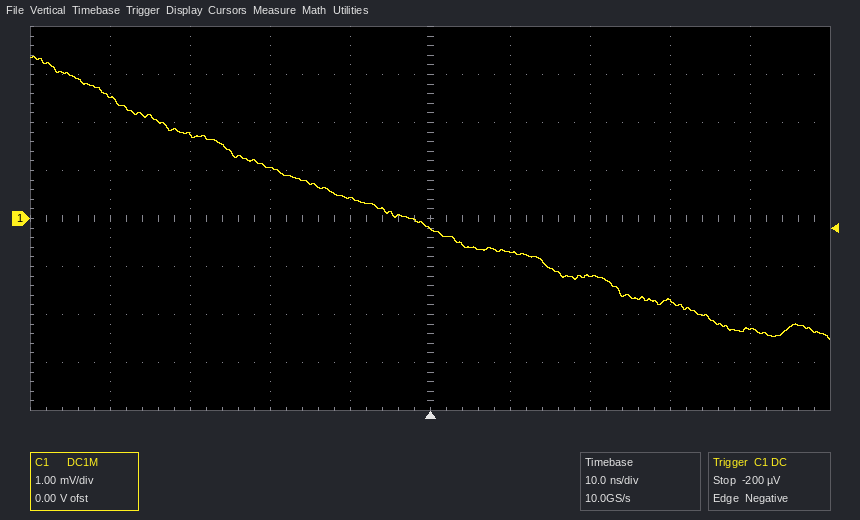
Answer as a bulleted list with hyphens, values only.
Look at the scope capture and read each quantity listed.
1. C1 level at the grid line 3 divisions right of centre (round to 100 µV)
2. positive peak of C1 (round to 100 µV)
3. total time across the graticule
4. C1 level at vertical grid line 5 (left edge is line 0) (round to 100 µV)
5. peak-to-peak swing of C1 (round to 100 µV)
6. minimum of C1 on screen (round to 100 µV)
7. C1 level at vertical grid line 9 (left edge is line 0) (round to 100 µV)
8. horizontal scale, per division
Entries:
- -1.7 mV
- 3.4 mV
- 100 ns
- -200 µV
- 5.9 mV
- -2.5 mV
- -2.3 mV
- 10 ns
